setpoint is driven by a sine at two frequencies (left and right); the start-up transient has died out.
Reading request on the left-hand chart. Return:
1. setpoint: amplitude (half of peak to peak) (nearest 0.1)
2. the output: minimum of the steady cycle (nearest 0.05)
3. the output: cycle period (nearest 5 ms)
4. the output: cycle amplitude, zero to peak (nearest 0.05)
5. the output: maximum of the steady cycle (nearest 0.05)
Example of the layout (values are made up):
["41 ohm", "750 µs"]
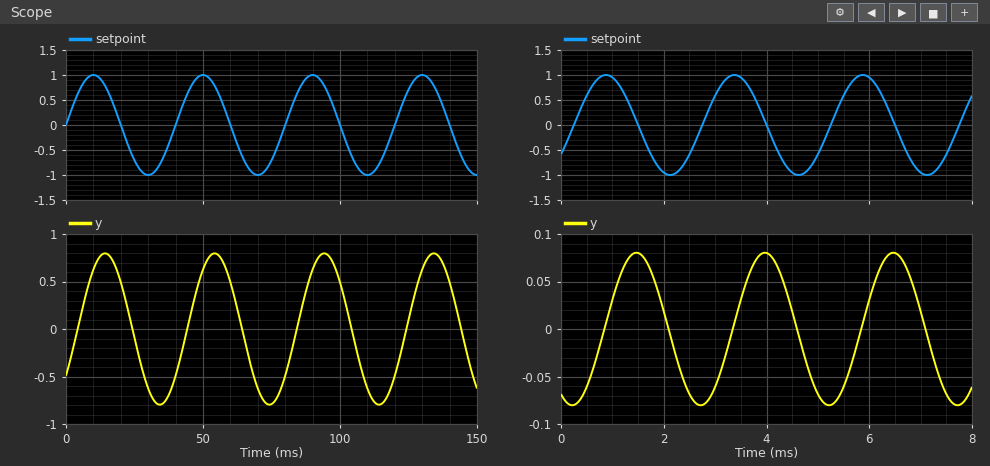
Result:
["1.0", "-0.80", "40 ms", "0.80", "0.80"]
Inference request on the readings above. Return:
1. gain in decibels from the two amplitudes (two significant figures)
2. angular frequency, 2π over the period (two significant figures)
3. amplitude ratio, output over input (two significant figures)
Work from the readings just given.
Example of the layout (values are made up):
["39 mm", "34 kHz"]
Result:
["-1.9 dB", "0.16 rad/ms", "0.80"]
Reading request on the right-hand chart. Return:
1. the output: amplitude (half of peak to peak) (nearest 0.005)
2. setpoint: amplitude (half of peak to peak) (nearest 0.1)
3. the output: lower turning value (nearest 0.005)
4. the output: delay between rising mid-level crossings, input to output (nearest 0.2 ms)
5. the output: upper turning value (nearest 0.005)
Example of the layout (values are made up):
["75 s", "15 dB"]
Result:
["0.080", "1.0", "-0.080", "0.6 ms", "0.080"]
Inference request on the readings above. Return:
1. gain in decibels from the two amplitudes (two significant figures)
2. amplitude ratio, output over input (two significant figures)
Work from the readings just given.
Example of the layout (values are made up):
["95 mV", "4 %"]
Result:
["-22 dB", "0.080"]
